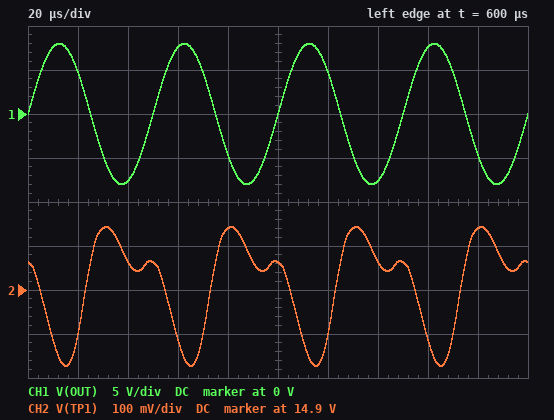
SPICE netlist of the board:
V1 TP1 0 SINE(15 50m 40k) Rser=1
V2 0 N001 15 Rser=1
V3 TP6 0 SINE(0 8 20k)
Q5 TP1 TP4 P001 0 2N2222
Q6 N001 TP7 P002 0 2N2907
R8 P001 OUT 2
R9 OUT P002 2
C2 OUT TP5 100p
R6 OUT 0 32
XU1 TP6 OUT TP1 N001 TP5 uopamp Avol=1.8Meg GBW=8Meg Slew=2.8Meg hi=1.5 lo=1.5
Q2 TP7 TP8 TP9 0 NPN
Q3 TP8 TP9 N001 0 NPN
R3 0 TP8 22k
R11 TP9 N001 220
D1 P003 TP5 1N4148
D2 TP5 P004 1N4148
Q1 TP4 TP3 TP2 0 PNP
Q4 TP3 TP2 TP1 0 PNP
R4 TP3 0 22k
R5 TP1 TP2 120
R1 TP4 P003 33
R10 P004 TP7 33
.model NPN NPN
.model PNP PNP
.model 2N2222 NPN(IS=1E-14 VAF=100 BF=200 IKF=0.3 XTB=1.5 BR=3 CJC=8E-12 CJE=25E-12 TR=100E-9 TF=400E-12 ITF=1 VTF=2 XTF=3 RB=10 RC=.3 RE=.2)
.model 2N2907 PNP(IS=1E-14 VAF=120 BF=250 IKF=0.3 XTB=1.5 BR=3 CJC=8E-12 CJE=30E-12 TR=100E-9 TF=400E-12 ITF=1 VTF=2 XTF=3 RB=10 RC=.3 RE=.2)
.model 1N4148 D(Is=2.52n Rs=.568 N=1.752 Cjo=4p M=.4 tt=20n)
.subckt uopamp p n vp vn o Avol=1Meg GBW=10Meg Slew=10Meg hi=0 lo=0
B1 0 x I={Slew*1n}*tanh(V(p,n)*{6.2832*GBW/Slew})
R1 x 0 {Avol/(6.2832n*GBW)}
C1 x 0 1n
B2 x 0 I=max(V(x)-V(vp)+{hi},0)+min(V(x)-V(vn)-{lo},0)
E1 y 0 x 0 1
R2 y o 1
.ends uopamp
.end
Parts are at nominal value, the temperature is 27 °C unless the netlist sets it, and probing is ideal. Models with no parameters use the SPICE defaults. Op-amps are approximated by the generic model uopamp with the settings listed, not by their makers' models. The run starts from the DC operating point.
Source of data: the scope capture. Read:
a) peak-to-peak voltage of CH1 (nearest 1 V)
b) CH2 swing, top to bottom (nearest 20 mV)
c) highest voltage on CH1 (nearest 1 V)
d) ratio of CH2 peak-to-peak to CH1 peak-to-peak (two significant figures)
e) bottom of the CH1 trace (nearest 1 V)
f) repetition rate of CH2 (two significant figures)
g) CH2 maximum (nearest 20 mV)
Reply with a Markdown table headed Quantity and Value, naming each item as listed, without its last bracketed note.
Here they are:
| Quantity | Value |
|---|---|
| peak-to-peak voltage of CH1 | 16 V |
| CH2 swing, top to bottom | 320 mV |
| highest voltage on CH1 | 8 V |
| ratio of CH2 peak-to-peak to CH1 peak-to-peak | 0.020 |
| bottom of the CH1 trace | -8 V |
| repetition rate of CH2 | 20 kHz |
| CH2 maximum | 15.04 V |
